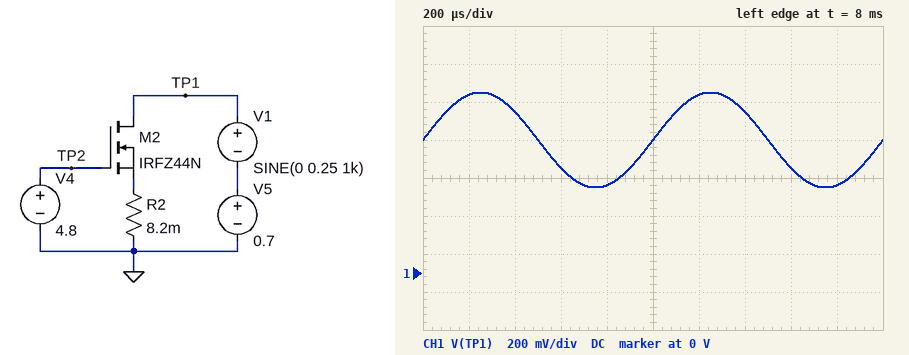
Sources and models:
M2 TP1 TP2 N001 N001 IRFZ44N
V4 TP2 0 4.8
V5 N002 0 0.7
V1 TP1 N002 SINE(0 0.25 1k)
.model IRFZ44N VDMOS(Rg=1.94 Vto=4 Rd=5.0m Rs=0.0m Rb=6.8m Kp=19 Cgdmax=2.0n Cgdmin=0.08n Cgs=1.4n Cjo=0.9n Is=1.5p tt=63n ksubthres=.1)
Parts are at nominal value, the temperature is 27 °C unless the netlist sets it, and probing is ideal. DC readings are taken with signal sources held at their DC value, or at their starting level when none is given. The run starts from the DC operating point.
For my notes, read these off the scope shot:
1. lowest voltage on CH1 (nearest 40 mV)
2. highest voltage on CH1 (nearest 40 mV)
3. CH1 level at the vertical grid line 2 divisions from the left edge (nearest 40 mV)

440 mV
960 mV
840 mV
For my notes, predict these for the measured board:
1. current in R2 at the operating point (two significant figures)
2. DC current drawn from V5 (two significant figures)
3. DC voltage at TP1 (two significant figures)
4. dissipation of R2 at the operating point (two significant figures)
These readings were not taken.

5.3 A
5.3 A
700 mV
230 mW
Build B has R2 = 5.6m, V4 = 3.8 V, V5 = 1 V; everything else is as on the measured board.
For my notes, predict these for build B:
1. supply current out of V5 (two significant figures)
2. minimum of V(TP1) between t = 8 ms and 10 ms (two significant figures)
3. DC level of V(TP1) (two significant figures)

1.5 mA
750 mV
1.0 V
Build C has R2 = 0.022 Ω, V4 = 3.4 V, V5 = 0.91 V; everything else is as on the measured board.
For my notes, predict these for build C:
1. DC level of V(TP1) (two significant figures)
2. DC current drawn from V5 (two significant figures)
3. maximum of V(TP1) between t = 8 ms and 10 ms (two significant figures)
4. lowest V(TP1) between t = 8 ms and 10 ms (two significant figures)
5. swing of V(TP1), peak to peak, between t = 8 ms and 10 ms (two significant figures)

910 mV
580 nA
1.2 V
660 mV
500 mV
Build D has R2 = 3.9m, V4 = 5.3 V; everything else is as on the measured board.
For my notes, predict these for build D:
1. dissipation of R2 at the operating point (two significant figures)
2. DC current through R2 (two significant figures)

470 mW
11 A
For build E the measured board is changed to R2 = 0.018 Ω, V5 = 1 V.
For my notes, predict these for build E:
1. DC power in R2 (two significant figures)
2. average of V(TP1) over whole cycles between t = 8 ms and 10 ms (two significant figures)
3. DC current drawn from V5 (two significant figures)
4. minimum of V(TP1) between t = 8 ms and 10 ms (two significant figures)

420 mW
1.0 V
4.8 A
750 mV
